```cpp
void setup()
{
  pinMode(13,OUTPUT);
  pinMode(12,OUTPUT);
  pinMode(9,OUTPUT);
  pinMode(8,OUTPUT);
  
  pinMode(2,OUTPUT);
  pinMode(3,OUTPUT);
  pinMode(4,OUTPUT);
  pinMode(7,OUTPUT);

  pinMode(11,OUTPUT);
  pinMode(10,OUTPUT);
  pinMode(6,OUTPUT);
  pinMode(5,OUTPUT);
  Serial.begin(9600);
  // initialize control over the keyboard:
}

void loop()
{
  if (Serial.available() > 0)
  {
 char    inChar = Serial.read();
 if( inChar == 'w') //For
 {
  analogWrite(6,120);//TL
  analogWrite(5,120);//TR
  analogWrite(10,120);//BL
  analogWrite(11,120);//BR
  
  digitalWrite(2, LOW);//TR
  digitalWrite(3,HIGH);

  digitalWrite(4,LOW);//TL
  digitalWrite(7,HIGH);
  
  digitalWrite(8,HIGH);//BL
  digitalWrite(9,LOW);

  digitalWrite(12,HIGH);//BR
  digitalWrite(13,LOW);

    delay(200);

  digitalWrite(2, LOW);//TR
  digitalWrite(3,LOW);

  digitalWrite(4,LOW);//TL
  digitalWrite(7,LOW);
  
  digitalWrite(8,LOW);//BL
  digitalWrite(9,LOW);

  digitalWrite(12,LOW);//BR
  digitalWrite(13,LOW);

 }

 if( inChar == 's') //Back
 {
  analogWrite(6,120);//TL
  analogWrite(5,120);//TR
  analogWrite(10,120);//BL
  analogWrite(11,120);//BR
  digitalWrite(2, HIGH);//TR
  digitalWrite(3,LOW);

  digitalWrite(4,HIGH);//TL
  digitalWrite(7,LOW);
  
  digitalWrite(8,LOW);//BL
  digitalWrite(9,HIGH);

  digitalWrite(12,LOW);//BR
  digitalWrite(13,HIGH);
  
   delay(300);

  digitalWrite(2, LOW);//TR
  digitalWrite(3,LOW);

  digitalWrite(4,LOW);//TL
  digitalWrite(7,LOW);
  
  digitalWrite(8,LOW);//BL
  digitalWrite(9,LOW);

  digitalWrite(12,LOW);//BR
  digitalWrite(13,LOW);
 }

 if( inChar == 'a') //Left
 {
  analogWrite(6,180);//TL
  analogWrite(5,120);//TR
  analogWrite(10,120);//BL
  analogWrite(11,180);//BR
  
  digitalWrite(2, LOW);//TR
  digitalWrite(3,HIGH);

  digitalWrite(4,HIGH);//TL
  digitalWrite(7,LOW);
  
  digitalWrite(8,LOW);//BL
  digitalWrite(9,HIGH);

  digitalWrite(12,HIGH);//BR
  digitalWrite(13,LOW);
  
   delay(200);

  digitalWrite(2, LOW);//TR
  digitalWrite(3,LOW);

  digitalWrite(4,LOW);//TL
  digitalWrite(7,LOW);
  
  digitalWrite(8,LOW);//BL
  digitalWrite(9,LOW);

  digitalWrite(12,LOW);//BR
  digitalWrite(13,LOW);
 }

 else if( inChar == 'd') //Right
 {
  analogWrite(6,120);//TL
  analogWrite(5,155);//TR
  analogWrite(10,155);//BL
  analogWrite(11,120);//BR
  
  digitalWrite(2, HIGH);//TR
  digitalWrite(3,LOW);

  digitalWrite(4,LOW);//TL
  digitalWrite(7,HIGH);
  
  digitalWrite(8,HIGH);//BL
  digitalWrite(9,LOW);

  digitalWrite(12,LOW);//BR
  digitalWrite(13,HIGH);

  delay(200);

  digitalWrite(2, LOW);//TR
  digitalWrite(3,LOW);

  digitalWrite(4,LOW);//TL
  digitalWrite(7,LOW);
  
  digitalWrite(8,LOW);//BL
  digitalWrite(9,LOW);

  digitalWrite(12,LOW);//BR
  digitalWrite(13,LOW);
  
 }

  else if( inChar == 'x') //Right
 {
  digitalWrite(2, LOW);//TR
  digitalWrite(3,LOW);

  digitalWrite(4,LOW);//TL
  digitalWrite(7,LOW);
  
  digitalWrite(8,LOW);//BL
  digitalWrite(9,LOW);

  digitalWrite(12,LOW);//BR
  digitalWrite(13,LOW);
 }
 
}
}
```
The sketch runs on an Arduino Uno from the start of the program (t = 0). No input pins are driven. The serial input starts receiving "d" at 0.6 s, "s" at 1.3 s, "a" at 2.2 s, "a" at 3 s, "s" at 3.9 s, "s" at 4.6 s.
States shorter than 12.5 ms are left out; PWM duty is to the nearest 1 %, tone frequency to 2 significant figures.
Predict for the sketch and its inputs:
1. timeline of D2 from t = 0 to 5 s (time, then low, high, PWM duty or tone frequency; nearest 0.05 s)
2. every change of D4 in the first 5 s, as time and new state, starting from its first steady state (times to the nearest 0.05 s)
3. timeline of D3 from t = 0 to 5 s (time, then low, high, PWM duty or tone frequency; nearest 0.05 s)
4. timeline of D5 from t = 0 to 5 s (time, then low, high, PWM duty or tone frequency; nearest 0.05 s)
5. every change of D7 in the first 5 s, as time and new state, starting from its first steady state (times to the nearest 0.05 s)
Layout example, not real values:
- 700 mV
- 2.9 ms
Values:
- 0 s low; 0.6 s high; 0.8 s low; 1.3 s high; 1.6 s low; 3.9 s high; 4.2 s low; 4.6 s high; 4.9 s low
- 0 s low; 1.3 s high; 1.6 s low; 2.2 s high; 2.4 s low; 3 s high; 3.2 s low; 3.9 s high; 4.2 s low; 4.6 s high; 4.9 s low
- 0 s low; 2.2 s high; 2.4 s low; 3 s high; 3.2 s low
- 0 s low; 0.6 s PWM 61 %; 1.3 s PWM 47 %
- 0 s low; 0.6 s high; 0.8 s low
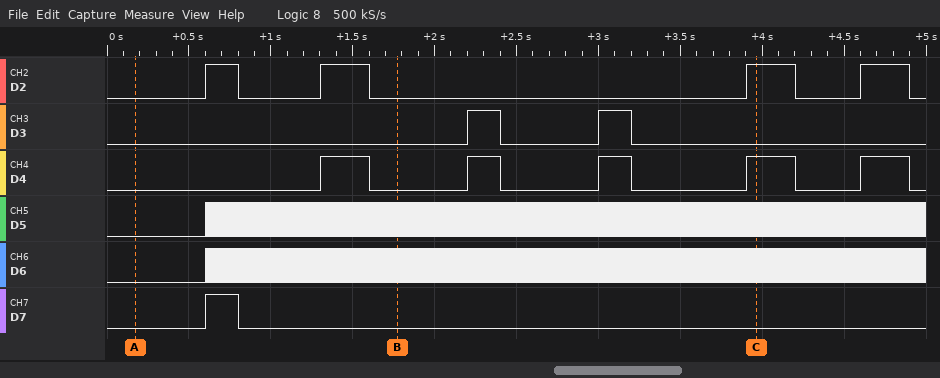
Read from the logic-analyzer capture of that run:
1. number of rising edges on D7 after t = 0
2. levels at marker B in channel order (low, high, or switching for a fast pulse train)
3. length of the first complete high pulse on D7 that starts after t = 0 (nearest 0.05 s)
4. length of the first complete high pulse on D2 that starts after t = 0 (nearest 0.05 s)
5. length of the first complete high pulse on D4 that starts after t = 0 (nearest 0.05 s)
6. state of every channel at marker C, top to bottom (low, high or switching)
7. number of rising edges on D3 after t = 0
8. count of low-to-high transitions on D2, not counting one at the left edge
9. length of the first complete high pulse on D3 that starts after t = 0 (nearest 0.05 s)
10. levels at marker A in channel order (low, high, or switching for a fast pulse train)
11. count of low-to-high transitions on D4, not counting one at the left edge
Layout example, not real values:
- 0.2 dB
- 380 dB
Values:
- 1
- D2 low, D3 low, D4 low, D5 switching, D6 switching, D7 low
- 0.20 s
- 0.20 s
- 0.30 s
- D2 high, D3 low, D4 high, D5 switching, D6 switching, D7 low
- 2
- 4
- 0.20 s
- D2 low, D3 low, D4 low, D5 low, D6 low, D7 low
- 5
